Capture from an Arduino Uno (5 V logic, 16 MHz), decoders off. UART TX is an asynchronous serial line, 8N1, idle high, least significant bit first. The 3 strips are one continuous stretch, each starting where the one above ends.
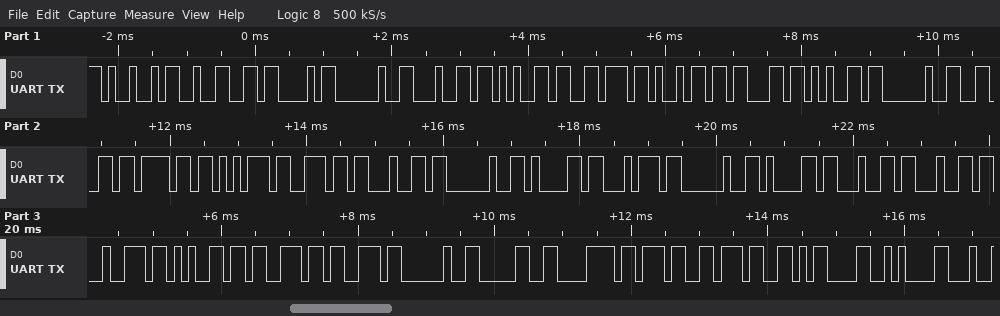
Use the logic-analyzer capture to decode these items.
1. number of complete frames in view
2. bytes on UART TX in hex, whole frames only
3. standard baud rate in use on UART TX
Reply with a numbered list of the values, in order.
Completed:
1. 34
2. 0x49 0x32 0x43 0x20 0x64 0x65 0x76 0x69 0x63 0x65 0x20 0x66 0x6F 0x75 0x6E 0x64 0x20 0x61 0x74 0x20 0x61 0x64 0x64 0x72 0x65 0x73 0x73 0x20 0x30 0x78 0x37 0x37 0x0D 0x0A
3. 9600 baud
